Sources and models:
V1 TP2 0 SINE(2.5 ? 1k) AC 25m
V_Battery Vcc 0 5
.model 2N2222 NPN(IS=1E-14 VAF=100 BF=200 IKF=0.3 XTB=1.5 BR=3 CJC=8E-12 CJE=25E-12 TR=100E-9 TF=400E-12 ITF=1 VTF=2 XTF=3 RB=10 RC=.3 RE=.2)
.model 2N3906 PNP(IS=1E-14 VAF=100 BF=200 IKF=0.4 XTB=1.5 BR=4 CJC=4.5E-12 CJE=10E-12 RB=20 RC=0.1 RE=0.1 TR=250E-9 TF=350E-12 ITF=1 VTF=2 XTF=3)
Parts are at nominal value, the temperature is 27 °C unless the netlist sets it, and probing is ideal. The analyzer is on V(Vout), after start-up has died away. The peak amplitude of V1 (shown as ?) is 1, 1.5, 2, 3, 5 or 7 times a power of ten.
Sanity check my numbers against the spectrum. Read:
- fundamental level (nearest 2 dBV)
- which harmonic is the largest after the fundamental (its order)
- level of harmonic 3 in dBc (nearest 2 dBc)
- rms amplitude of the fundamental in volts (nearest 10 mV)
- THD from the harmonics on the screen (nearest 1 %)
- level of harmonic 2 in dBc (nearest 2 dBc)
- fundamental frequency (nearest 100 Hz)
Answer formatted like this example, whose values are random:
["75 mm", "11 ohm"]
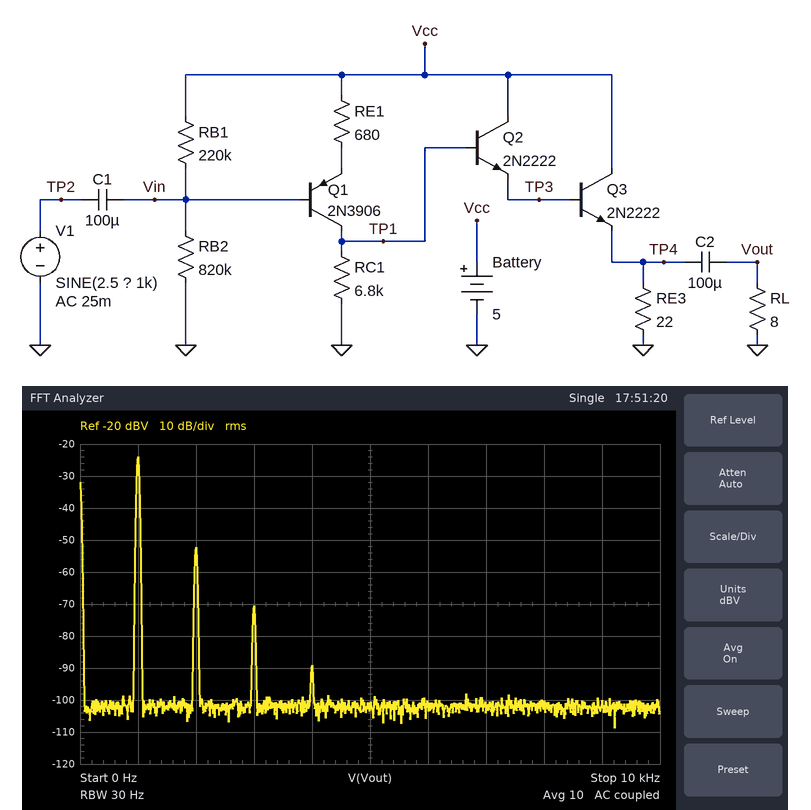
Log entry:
["-24 dBV", "2", "-46 dBc", "60 mV", "4 %", "-28 dBc", "1.0 kHz"]
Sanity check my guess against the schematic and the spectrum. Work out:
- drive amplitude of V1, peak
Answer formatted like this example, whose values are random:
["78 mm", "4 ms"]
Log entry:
["15 mV"]
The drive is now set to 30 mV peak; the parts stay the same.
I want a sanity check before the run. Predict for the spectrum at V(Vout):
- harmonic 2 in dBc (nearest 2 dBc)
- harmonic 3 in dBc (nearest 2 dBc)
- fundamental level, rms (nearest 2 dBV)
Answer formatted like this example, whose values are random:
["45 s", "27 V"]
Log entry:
["-20 dBc", "-32 dBc", "-18 dBV"]
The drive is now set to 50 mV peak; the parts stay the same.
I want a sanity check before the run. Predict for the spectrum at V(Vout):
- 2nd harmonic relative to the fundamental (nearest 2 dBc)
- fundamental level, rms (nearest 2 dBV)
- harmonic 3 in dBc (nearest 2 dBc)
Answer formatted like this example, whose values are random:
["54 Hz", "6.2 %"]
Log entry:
["-12 dBc", "-16 dBV", "-26 dBc"]
